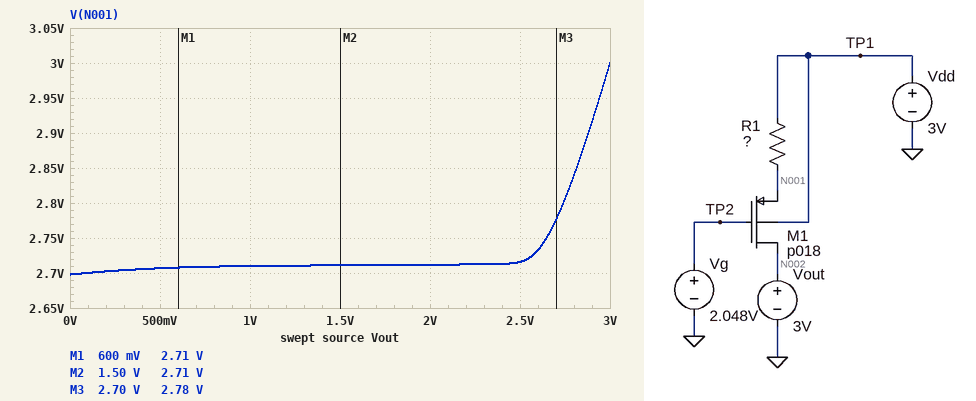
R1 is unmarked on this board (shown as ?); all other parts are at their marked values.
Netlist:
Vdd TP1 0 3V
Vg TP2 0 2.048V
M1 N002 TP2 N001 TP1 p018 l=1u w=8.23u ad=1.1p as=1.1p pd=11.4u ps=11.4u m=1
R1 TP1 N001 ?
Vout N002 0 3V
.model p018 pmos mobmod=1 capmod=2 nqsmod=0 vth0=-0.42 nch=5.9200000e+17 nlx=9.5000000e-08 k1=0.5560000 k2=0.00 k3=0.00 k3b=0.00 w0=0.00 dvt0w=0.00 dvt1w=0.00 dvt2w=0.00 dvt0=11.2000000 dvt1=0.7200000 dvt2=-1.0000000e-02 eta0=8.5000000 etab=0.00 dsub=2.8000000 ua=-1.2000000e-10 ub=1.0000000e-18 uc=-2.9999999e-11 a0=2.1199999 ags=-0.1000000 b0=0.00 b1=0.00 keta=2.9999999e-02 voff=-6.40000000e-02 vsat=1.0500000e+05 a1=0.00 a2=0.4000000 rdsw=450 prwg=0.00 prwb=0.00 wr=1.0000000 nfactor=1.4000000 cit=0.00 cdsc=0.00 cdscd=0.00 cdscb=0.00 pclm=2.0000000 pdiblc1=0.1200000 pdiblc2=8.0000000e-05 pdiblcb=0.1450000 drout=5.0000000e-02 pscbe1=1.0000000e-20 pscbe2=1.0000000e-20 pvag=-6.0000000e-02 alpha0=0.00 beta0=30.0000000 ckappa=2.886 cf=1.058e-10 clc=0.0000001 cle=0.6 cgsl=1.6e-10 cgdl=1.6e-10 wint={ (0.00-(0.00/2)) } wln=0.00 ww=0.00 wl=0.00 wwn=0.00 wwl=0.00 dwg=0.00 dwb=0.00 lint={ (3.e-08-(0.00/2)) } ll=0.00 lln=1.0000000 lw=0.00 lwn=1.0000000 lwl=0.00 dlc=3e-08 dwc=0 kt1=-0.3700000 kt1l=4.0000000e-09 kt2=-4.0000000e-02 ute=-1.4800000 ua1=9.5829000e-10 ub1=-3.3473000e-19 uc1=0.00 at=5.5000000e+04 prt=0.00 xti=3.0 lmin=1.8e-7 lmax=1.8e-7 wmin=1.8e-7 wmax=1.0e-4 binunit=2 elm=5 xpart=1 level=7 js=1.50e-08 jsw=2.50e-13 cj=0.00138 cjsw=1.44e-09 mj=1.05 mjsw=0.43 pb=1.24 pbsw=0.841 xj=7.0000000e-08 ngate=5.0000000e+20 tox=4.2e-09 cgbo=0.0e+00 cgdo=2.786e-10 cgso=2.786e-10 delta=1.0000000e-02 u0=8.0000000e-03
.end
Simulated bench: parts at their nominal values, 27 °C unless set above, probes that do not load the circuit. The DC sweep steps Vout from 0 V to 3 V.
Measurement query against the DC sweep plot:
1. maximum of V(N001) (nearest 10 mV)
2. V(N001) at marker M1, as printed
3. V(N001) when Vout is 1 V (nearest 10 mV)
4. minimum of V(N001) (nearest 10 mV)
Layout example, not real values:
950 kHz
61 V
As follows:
3.00 V
2.71 V
2.71 V
2.70 V
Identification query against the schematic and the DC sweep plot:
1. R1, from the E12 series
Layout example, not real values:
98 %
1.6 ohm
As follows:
39 kΩ
